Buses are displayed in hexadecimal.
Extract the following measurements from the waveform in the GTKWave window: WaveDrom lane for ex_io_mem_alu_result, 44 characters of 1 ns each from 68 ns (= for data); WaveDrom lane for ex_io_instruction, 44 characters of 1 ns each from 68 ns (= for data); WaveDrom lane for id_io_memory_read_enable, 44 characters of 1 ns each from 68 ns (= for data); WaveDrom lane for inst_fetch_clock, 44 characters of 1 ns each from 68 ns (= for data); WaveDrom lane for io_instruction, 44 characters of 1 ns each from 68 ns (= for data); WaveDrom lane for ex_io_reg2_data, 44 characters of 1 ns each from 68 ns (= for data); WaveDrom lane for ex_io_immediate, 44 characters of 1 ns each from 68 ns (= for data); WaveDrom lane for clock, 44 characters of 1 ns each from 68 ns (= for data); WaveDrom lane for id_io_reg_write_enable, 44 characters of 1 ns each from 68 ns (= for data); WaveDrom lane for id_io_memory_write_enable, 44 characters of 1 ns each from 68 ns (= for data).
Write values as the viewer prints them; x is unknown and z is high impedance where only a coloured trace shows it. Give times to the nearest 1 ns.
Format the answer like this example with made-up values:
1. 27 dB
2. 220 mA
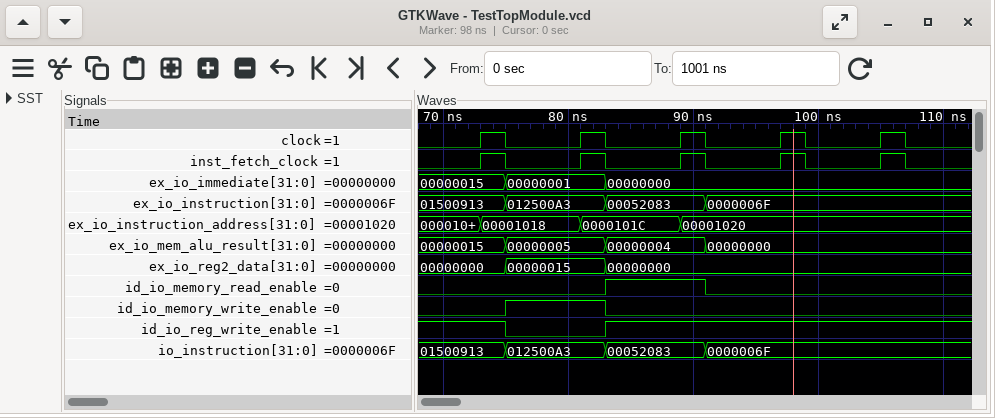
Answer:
1. {name: 'ex_io_mem_alu_result', wave: '=......=.......=.......=....................', data: '00000015 00000005 00000004 00000000'}
2. {name: 'ex_io_instruction', wave: '=......=.......=.......=....................', data: '01500913 012500A3 00052083 0000006F'}
3. {name: 'id_io_memory_read_enable', wave: '0..............1.......0....................'}
4. {name: 'inst_fetch_clock', wave: '0....1.0.....1.0.....1.0.....1.0.....1.0....'}
5. {name: 'io_instruction', wave: '=......=.......=.......=....................', data: '01500913 012500A3 00052083 0000006F'}
6. {name: 'ex_io_reg2_data', wave: '=......=.......=............................', data: '00000000 00000015 00000000'}
7. {name: 'ex_io_immediate', wave: '=......=.......=............................', data: '00000015 00000001 00000000'}
8. {name: 'clock', wave: '0....1.0.....1.0.....1.0.....1.0.....1.0....'}
9. {name: 'id_io_reg_write_enable', wave: '1......0.......1............................'}
10. {name: 'id_io_memory_write_enable', wave: '0......1.......0............................'}
